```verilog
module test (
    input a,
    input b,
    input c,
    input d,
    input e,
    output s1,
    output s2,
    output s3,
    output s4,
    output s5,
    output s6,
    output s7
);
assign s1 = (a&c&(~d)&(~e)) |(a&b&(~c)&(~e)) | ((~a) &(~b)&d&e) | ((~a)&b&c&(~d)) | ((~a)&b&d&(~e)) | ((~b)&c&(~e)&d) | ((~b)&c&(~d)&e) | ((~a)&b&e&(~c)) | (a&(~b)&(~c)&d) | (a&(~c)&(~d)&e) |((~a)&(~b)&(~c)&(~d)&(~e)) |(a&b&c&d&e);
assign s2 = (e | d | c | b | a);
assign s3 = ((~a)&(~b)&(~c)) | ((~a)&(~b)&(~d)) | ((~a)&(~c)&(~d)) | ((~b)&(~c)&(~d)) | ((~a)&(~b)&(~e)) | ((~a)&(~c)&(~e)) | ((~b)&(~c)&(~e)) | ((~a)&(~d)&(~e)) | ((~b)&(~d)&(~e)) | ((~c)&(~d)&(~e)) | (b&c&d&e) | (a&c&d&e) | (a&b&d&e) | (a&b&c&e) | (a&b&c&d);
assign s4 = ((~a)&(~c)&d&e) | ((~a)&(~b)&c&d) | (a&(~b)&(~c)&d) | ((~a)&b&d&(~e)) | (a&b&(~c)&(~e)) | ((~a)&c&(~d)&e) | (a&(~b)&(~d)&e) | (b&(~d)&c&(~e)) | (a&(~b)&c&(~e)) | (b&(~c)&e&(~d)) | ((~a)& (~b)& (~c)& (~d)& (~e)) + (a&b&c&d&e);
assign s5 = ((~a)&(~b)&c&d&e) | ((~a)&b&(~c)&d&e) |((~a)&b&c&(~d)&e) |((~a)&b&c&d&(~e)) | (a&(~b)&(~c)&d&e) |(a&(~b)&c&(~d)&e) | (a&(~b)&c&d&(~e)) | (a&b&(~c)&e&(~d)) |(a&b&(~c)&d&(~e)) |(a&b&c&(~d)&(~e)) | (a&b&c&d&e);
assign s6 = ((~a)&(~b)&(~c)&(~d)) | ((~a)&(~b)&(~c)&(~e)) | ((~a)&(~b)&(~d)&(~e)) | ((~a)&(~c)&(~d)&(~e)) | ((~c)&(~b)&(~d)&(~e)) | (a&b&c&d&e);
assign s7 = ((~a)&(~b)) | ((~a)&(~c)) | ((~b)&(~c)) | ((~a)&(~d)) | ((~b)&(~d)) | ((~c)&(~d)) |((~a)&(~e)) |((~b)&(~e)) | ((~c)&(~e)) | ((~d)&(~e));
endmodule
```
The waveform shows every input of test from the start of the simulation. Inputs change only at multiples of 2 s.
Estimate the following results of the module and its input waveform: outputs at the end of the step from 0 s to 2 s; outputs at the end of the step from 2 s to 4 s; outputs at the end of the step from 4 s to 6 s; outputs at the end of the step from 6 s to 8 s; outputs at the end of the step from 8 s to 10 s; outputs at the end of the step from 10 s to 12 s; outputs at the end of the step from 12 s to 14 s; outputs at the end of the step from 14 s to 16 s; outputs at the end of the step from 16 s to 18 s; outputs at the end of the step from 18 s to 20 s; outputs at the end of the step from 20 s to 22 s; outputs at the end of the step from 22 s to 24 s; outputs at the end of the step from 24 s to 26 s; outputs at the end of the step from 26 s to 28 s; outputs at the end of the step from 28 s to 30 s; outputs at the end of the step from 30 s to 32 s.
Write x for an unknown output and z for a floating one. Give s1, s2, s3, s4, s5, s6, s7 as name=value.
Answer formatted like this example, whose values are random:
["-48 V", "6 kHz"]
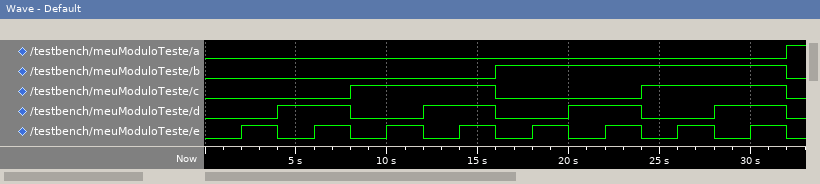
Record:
["s1=1, s2=0, s3=1, s4=1, s5=0, s6=1, s7=1", "s1=0, s2=1, s3=1, s4=0, s5=0, s6=1, s7=1", "s1=0, s2=1, s3=1, s4=0, s5=0, s6=1, s7=1", "s1=1, s2=1, s3=1, s4=1, s5=0, s6=0, s7=1", "s1=0, s2=1, s3=1, s4=0, s5=0, s6=1, s7=1", "s1=1, s2=1, s3=1, s4=1, s5=0, s6=0, s7=1", "s1=1, s2=1, s3=1, s4=1, s5=0, s6=0, s7=1", "s1=1, s2=1, s3=0, s4=1, s5=1, s6=0, s7=1", "s1=0, s2=1, s3=1, s4=0, s5=0, s6=1, s7=1", "s1=1, s2=1, s3=1, s4=1, s5=0, s6=0, s7=1", "s1=1, s2=1, s3=1, s4=1, s5=0, s6=0, s7=1", "s1=1, s2=1, s3=0, s4=1, s5=1, s6=0, s7=1", "s1=1, s2=1, s3=1, s4=1, s5=0, s6=0, s7=1", "s1=1, s2=1, s3=0, s4=1, s5=1, s6=0, s7=1", "s1=1, s2=1, s3=0, s4=1, s5=1, s6=0, s7=1", "s1=0, s2=1, s3=1, s4=0, s5=0, s6=0, s7=0"]
